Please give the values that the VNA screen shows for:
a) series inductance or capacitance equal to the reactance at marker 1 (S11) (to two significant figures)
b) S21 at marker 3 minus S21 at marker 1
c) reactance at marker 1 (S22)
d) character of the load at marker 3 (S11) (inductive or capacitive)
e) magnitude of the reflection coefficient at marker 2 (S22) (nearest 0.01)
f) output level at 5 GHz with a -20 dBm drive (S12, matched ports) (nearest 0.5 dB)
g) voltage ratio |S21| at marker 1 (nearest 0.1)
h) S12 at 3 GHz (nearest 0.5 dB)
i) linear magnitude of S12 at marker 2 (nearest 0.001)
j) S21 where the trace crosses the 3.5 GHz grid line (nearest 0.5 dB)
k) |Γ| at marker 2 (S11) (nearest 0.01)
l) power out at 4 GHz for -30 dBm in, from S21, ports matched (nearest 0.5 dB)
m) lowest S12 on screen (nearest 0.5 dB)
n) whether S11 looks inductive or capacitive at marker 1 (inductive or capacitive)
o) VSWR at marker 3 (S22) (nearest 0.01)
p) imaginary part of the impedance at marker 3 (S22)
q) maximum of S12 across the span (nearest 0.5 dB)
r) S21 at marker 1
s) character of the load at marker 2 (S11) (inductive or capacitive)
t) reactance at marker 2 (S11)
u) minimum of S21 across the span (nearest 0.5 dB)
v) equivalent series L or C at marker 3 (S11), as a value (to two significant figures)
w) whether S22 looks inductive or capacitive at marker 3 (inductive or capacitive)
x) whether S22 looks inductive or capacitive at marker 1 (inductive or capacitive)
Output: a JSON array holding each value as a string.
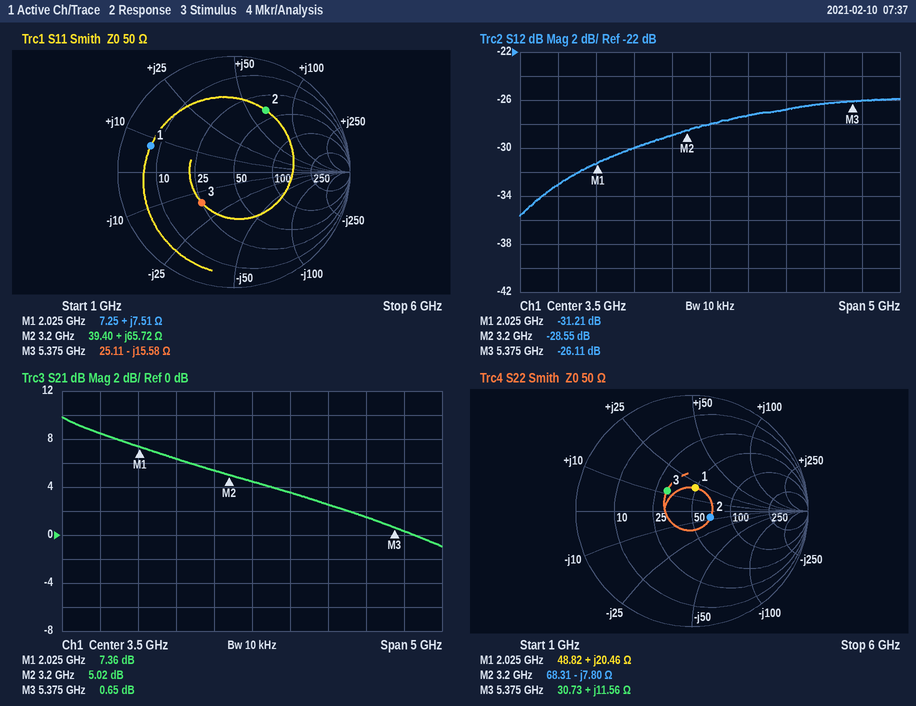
["590 pH", "-6.71 dB", "+20.46 Ω", "capacitive", "0.17", "-46.5 dBm", "2.3", "-29.0 dB", "0.037", "4.5 dB", "0.60", "-26.5 dBm", "-35.5 dB", "inductive", "1.76", "+11.56 Ω", "-26.0 dB", "7.36 dB", "inductive", "+65.72 Ω", "-1.0 dB", "1.9 pF", "inductive", "inductive"]
